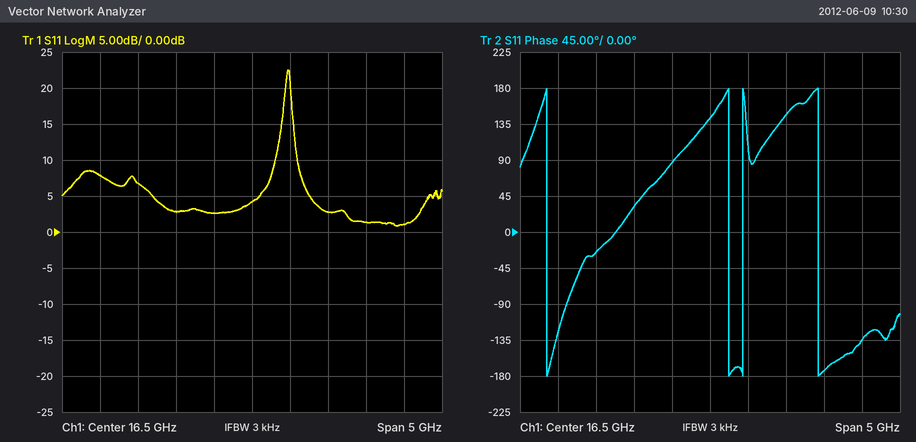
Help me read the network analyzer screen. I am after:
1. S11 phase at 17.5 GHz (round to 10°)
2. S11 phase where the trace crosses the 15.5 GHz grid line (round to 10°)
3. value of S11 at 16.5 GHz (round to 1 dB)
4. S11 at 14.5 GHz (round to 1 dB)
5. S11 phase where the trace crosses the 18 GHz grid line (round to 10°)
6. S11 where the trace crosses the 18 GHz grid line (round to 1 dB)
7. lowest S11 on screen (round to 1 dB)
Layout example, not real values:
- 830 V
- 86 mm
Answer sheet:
- 150°
- 30°
- 4 dB
- 8 dB
- -170°
- 1 dB
- 1 dB
